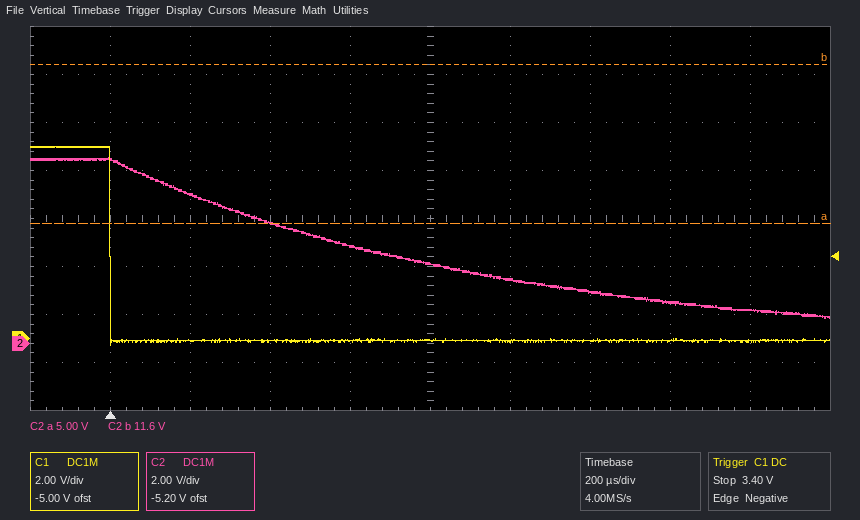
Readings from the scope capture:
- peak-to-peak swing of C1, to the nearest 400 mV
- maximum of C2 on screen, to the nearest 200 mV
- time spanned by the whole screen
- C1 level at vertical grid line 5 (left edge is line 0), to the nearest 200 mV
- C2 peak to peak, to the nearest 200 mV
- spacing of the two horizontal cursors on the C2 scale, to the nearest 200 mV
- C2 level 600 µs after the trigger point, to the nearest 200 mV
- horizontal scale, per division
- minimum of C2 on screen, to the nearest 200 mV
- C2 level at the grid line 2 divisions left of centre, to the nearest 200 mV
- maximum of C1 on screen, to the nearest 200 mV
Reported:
8.4 V
7.8 V
2 ms
0.0 V
6.8 V
6.6 V
4.0 V
200 µs
1.0 V
5.0 V
8.0 V
